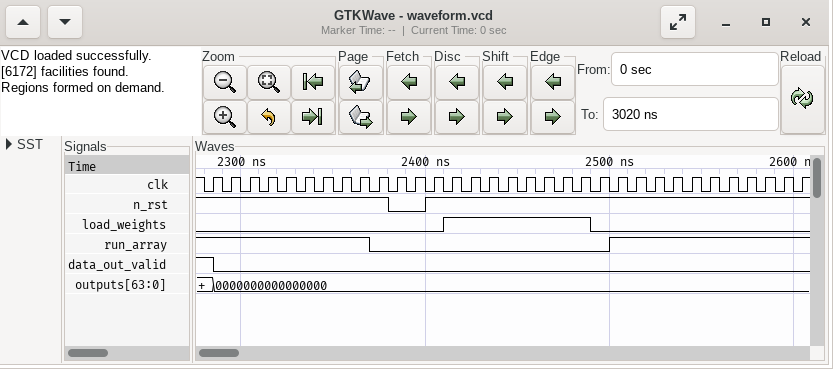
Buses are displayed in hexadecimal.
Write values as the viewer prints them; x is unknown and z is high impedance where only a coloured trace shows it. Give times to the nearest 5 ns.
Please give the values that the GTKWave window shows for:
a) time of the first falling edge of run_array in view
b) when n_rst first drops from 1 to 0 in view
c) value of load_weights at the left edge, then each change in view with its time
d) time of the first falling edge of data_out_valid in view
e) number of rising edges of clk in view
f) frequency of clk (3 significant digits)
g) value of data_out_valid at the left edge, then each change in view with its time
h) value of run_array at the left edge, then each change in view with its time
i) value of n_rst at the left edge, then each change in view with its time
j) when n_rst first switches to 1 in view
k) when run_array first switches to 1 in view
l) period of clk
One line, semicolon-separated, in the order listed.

2370 ns; 2380 ns; 0, 1 at 2410 ns, 0 at 2490 ns; 2285 ns; 33; 100 MHz; 1, 0 at 2285 ns; 1, 0 at 2370 ns, 1 at 2500 ns; 1, 0 at 2380 ns, 1 at 2400 ns; 2400 ns; 2500 ns; 10 ns
